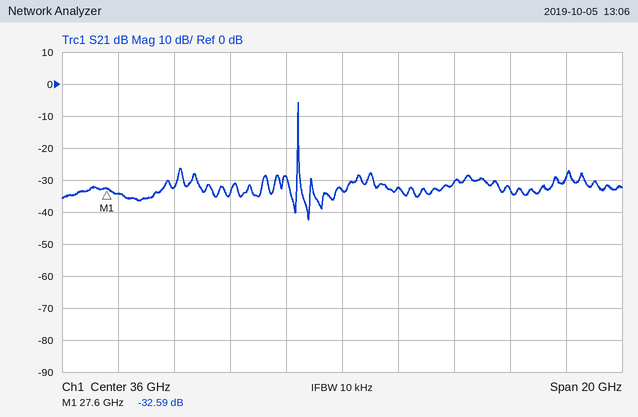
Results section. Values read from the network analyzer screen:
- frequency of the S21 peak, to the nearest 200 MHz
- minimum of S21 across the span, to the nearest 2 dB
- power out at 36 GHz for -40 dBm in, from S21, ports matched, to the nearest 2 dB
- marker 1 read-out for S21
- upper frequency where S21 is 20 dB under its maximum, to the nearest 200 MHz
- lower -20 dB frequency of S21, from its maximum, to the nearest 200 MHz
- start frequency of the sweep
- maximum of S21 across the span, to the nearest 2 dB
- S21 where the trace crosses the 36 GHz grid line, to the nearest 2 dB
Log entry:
34.4 GHz
-42 dB
-74 dBm
-32.59 dB
34.4 GHz
34.4 GHz
26 GHz
-6 dB
-34 dB
